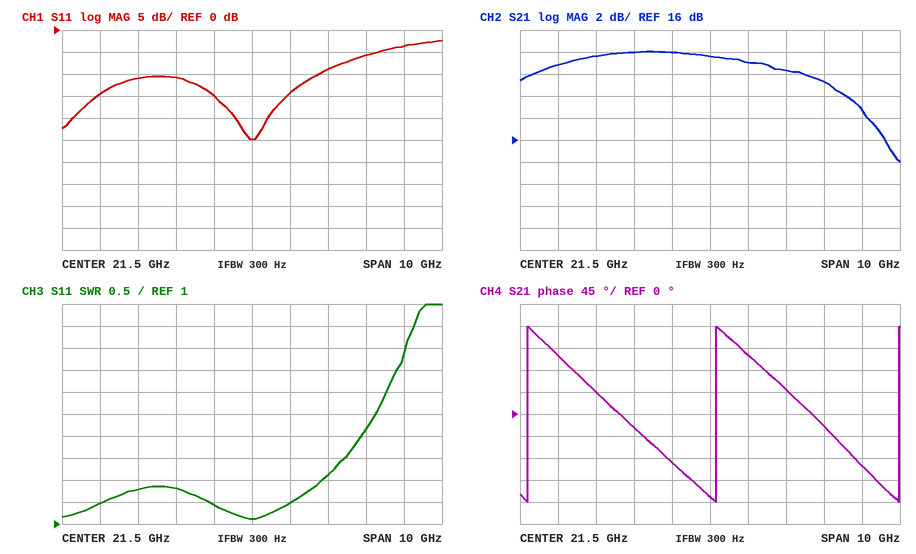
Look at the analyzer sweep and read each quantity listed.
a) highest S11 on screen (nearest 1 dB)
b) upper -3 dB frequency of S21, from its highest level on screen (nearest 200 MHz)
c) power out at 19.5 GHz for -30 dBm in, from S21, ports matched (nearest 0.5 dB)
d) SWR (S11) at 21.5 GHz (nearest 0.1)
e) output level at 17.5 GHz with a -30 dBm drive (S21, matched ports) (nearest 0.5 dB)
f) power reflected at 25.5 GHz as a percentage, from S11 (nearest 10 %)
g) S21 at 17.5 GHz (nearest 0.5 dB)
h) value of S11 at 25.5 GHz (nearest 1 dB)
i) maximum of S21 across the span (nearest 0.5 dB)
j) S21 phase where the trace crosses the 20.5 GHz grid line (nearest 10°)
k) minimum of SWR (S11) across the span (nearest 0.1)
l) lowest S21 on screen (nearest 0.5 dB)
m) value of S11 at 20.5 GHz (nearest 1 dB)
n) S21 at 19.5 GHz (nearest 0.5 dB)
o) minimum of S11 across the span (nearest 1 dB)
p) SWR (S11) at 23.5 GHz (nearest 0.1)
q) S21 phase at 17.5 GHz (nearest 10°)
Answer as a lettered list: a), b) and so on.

a) -2 dB
b) 24.6 GHz
c) -6.0 dBm
d) 1.1
e) -7.0 dBm
f) 40 %
g) 23.0 dB
h) -4 dB
i) 24.0 dB
j) -100°
k) 1.1
l) 14.0 dB
m) -15 dB
n) 24.0 dB
o) -25 dB
p) 2.1
q) 120°
